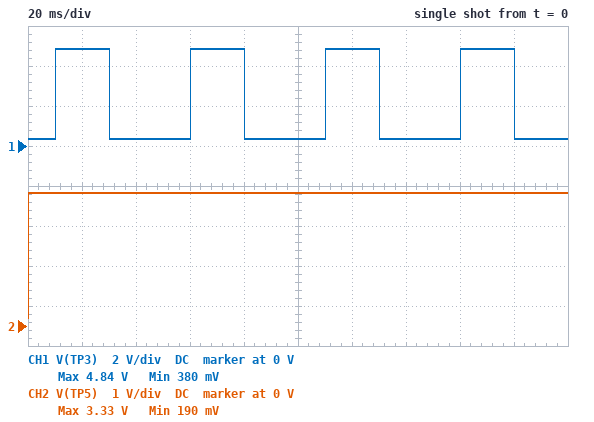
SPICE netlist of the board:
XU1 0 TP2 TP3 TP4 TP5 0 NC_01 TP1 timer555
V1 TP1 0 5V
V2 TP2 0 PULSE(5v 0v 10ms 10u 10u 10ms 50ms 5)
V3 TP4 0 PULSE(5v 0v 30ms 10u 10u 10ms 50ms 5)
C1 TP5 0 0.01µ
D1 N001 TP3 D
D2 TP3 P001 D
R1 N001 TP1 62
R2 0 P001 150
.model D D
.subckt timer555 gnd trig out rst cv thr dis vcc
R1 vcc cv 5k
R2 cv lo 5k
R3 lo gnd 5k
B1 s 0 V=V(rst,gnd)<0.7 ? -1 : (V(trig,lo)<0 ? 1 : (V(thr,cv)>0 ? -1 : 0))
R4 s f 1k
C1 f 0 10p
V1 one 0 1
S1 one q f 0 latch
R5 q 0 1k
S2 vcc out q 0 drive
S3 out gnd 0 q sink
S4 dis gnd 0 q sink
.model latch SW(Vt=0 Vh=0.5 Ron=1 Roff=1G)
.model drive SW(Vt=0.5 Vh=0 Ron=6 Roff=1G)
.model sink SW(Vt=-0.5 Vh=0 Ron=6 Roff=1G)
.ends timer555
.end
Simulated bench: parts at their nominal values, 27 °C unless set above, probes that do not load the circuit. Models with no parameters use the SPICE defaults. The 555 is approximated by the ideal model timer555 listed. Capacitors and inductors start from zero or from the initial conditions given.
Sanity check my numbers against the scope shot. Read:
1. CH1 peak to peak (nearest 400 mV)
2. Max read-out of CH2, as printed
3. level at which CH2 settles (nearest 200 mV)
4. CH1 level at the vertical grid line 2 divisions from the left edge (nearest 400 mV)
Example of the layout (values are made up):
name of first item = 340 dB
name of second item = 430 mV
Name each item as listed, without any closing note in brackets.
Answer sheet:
CH1 peak to peak = 4.4 V
Max read-out of CH2, as printed = 3.33 V
level at which CH2 settles = 3.4 V
CH1 level at the vertical grid line 2 divisions from the left edge = 400 mV
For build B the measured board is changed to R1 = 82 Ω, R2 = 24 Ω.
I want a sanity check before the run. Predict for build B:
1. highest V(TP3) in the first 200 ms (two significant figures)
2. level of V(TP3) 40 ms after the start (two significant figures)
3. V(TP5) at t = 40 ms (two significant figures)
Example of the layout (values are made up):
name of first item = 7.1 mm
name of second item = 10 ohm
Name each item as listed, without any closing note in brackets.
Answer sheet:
highest V(TP3) in the first 200 ms = 4.2 V
level of V(TP3) 40 ms after the start = 290 mV
V(TP5) at t = 40 ms = 3.3 V
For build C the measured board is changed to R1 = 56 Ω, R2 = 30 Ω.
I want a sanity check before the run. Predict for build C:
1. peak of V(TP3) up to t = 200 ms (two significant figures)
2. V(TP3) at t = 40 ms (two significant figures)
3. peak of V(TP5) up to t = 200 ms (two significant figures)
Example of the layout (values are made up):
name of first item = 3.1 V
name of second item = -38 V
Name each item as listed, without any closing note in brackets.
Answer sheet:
peak of V(TP3) up to t = 200 ms = 4.3 V
V(TP3) at t = 40 ms = 410 mV
peak of V(TP5) up to t = 200 ms = 3.3 V
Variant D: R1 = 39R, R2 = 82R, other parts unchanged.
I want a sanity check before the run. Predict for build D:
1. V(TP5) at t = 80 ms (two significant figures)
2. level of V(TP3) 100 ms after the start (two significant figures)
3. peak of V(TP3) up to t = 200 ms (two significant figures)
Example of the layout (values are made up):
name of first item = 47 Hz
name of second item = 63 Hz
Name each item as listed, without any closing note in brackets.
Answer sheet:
V(TP5) at t = 80 ms = 3.3 V
level of V(TP3) 100 ms after the start = 560 mV
peak of V(TP3) up to t = 200 ms = 4.7 V
